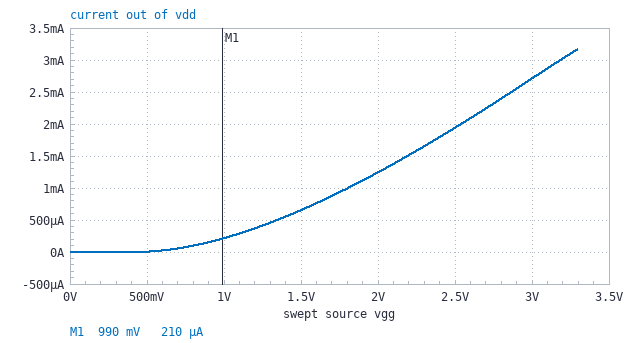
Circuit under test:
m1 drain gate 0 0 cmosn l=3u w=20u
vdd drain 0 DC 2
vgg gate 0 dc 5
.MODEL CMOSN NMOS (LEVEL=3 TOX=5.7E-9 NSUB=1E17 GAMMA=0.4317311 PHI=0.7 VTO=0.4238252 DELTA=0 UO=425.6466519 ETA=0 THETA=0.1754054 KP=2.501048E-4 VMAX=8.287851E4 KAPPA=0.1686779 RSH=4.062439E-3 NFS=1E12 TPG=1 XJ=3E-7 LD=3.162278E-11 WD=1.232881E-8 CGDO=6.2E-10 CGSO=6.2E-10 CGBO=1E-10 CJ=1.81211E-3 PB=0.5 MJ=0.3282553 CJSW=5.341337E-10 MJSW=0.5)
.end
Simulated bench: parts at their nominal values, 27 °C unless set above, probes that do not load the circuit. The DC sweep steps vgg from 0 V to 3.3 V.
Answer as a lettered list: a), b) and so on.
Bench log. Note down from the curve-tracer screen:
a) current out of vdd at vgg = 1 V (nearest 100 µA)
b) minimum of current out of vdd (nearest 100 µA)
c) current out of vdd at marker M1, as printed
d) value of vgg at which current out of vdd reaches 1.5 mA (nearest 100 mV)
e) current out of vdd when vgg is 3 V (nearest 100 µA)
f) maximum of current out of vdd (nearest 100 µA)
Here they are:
a) 200 µA
b) 0 A
c) 210 µA
d) 2.2 V
e) 2.7 mA
f) 3.2 mA
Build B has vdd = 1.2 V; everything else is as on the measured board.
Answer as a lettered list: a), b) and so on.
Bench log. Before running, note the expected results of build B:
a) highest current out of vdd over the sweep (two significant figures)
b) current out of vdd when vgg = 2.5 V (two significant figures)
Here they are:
a) 2.6 mA
b) 1.8 mA
